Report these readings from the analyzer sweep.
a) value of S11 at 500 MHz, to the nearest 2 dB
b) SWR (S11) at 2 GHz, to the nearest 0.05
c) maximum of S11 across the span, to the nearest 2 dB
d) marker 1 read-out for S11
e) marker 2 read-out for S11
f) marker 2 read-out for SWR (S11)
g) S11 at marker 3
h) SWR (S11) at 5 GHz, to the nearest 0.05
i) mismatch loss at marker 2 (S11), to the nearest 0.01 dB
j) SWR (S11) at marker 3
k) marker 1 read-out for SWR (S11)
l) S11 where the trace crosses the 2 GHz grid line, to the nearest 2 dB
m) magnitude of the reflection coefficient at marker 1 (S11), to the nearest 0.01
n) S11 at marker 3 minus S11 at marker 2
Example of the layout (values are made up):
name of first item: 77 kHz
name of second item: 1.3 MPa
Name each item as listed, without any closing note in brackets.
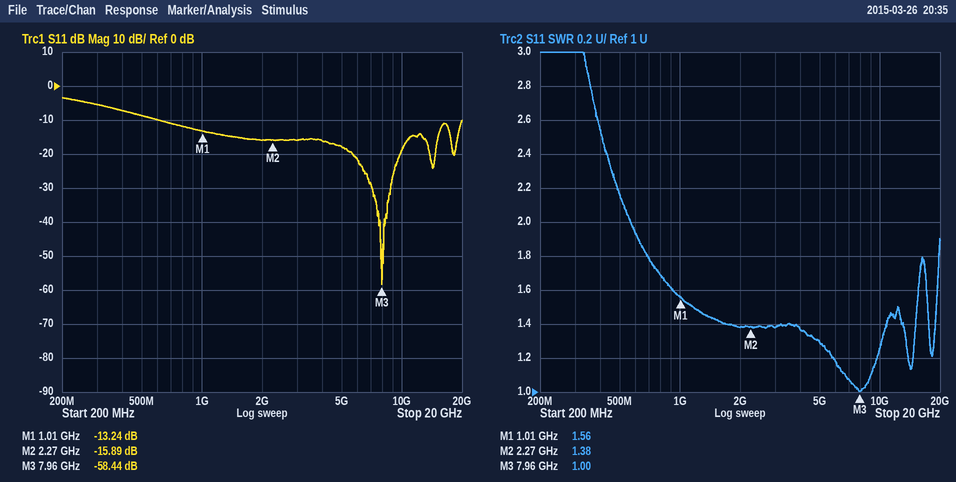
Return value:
value of S11 at 500 MHz, to the nearest 2 dB: -8 dB
SWR (S11) at 2 GHz, to the nearest 0.05: 1.40
maximum of S11 across the span, to the nearest 2 dB: -4 dB
marker 1 read-out for S11: -13.24 dB
marker 2 read-out for S11: -15.89 dB
marker 2 read-out for SWR: 1.38
S11 at marker 3: -58.44 dB
SWR (S11) at 5 GHz, to the nearest 0.05: 1.30
mismatch loss at marker 2 (S11), to the nearest 0.01 dB: 0.11 dB
SWR (S11) at marker 3: 1.00
marker 1 read-out for SWR: 1.56
S11 where the trace crosses the 2 GHz grid line, to the nearest 2 dB: -16 dB
magnitude of the reflection coefficient at marker 1 (S11), to the nearest 0.01: 0.22
S11 at marker 3 minus S11 at marker 2: -42.55 dB
